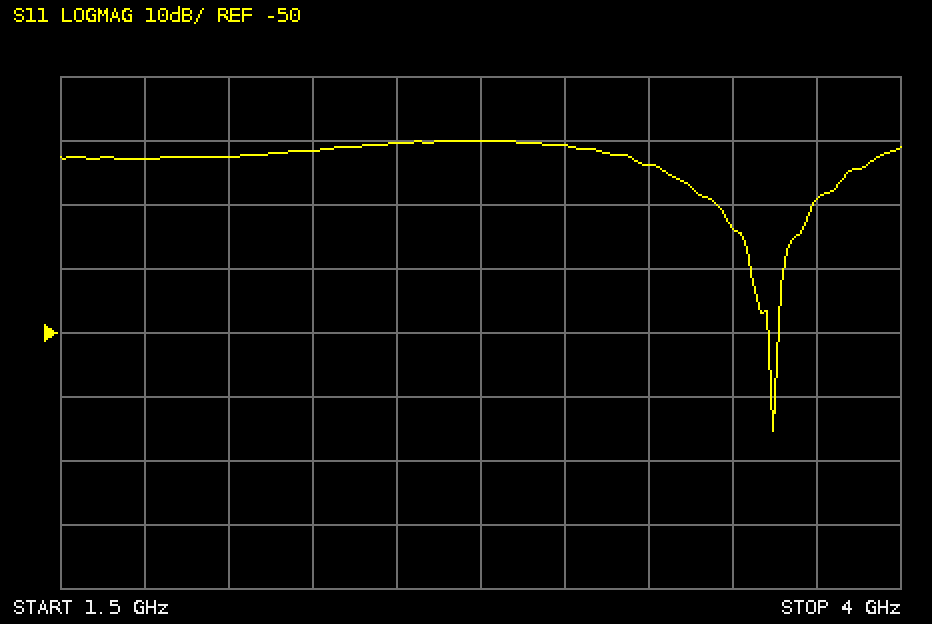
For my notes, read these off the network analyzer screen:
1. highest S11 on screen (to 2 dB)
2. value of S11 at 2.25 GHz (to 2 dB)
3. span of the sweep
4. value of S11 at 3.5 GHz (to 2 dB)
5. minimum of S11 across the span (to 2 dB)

-20 dB
-22 dB
2.5 GHz
-34 dB
-66 dB
